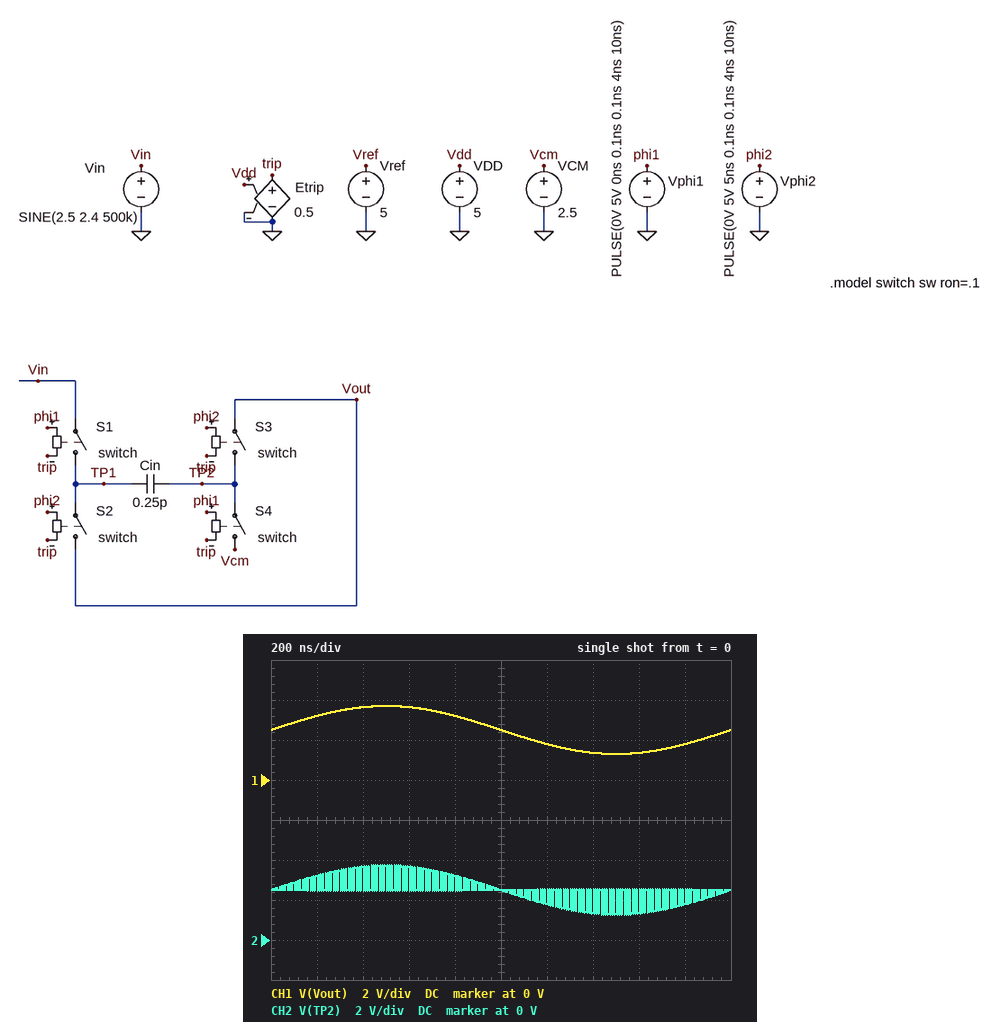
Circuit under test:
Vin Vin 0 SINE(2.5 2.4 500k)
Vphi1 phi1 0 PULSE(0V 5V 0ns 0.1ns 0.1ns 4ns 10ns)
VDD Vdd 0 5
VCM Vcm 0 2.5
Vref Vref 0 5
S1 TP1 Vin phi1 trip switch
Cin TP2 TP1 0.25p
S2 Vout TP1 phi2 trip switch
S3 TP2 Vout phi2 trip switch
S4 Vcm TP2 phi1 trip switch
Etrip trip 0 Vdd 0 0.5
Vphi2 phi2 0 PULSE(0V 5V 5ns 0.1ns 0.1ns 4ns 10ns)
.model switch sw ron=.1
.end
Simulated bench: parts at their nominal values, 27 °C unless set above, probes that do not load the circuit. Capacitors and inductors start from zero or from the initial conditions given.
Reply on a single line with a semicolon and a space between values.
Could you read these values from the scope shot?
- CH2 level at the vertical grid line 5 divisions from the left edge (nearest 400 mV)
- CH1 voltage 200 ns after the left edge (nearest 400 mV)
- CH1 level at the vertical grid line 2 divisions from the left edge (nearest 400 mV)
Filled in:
2.4 V; 3.2 V; 3.6 V
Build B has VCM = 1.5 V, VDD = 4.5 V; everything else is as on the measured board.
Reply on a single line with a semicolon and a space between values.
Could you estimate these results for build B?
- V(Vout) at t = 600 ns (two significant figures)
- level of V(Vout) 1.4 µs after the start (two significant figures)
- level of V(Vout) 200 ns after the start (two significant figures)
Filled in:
3.1 V; 860 mV; 2.7 V
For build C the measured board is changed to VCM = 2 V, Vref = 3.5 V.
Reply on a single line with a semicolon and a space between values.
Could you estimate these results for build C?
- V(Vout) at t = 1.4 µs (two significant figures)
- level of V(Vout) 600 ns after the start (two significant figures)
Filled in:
1.1 V; 3.4 V
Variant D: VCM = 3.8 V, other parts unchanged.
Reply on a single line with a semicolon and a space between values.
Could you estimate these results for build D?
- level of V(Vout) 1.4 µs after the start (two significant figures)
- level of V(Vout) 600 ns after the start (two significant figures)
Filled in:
2.0 V; 4.3 V
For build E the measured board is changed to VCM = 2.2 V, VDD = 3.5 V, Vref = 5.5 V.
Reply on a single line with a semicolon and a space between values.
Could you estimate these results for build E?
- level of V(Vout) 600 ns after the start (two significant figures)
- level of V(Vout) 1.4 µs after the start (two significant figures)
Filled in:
3.5 V; 1.2 V
